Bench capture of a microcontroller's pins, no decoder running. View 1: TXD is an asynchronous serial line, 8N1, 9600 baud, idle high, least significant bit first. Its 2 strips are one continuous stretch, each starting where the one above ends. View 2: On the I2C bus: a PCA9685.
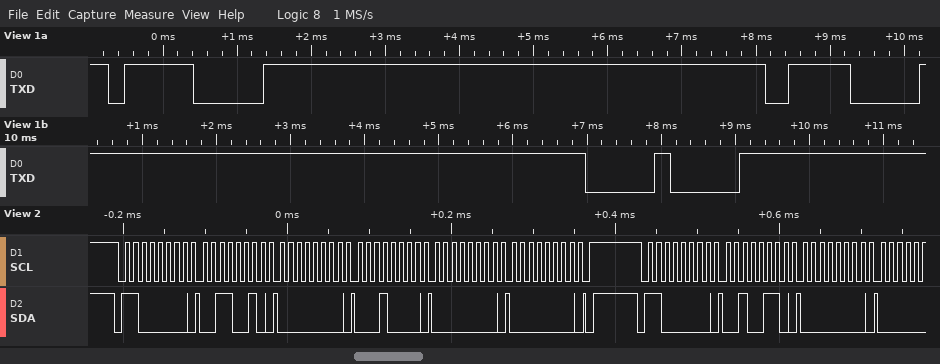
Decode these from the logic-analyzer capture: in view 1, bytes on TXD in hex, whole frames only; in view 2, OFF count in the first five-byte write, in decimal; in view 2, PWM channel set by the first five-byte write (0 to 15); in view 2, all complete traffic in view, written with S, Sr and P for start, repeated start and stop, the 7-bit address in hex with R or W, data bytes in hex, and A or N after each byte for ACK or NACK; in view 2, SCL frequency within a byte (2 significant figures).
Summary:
0xFE 0x00 0xFC 0x00 0x00 0x00
0
11
S 60W A 32 A 00 A 10 A 00 A 00 A P S 60W A 26 A 00 A
100 kHz
